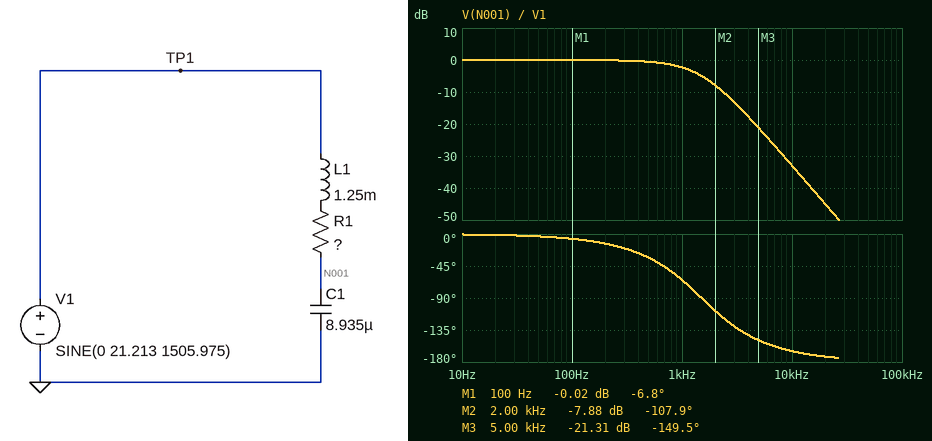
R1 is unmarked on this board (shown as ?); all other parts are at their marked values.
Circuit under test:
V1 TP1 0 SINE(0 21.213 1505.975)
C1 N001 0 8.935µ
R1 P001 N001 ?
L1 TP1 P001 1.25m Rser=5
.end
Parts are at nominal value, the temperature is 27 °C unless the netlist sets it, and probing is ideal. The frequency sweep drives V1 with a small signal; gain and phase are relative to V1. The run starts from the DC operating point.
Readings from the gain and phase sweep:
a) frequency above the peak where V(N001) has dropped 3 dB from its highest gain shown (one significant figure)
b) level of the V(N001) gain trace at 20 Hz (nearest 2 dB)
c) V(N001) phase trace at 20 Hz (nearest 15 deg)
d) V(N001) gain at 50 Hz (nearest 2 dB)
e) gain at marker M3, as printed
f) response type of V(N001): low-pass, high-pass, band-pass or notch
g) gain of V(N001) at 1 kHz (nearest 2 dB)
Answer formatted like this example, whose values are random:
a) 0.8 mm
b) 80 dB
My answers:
a) 1 kHz
b) 0 dB
c) 0 deg
d) 0 dB
e) -21.31 dB
f) low-pass
g) -2 dB
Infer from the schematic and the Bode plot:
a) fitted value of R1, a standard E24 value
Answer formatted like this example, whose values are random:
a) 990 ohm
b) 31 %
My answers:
a) 16 Ω
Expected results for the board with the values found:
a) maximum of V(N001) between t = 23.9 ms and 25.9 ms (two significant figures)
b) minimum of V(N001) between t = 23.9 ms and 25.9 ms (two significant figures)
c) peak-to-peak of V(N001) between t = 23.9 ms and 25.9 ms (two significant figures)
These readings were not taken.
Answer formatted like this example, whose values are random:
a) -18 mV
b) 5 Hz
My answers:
a) 12 V
b) -12 V
c) 24 V
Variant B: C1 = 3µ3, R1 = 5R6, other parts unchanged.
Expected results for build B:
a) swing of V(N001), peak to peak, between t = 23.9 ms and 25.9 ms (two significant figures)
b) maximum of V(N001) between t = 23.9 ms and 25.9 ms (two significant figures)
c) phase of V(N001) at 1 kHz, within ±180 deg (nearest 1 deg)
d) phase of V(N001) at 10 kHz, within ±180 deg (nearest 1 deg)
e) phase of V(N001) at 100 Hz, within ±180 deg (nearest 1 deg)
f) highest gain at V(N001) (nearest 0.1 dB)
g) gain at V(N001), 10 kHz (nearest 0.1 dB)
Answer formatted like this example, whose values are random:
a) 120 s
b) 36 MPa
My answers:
a) 60 V
b) 30 V
c) -15 deg
d) -172 deg
e) -1 deg
f) 5.6 dB
g) -23.8 dB
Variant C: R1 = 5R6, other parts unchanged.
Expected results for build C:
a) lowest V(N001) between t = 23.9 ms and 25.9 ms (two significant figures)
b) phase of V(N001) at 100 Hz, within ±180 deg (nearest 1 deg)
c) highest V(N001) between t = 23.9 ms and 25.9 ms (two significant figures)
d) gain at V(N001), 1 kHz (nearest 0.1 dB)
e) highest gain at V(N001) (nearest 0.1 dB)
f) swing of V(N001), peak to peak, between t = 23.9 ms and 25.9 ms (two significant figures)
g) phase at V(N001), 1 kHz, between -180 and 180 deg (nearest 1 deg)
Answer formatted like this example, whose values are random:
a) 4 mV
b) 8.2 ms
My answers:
a) -24 V
b) -3 deg
c) 24 V
d) 1.8 dB
e) 1.9 dB
f) 47 V
g) -47 deg
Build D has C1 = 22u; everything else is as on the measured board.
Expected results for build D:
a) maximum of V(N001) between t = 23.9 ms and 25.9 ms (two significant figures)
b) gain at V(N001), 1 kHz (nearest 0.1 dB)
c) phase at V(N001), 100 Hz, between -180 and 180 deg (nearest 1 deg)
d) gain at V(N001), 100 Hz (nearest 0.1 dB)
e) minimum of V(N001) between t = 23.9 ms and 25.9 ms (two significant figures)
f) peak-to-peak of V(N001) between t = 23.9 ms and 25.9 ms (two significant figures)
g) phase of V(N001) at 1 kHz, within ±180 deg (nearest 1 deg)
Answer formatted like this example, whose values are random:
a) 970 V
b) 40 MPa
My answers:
a) 4.6 V
b) -9.3 dB
c) -16 deg
d) -0.3 dB
e) -4.6 V
f) 9.2 V
g) -92 deg
